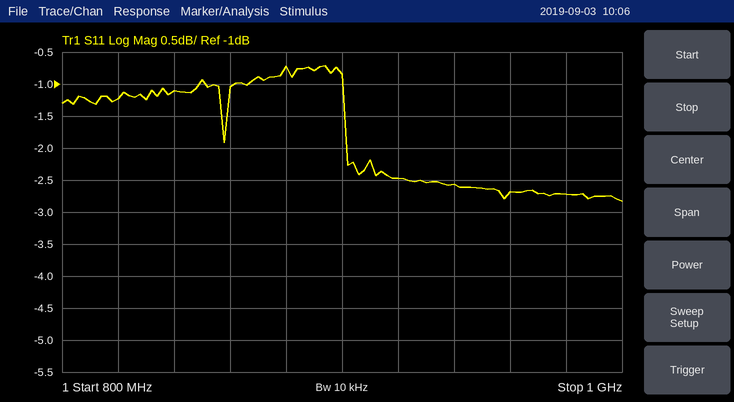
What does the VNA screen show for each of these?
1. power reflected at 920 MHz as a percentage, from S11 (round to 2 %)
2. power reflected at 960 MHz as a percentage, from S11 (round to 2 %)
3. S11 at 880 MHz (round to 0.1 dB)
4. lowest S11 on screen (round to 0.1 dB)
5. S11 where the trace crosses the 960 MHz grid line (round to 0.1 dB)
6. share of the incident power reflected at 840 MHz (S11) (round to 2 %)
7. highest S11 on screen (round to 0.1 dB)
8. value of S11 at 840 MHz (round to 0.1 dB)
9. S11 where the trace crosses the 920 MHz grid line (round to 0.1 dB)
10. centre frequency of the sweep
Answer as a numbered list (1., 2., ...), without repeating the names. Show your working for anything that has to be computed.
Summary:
1. 10^(-2.5/10) ≈ 56 %
2. 10^(-2.7/10) ≈ 54 %
3. -0.7 dB
4. -2.8 dB
5. -2.7 dB
6. 10^(-1.1/10) ≈ 78 %
7. -0.7 dB
8. -1.1 dB
9. -2.5 dB
10. 900 MHz
